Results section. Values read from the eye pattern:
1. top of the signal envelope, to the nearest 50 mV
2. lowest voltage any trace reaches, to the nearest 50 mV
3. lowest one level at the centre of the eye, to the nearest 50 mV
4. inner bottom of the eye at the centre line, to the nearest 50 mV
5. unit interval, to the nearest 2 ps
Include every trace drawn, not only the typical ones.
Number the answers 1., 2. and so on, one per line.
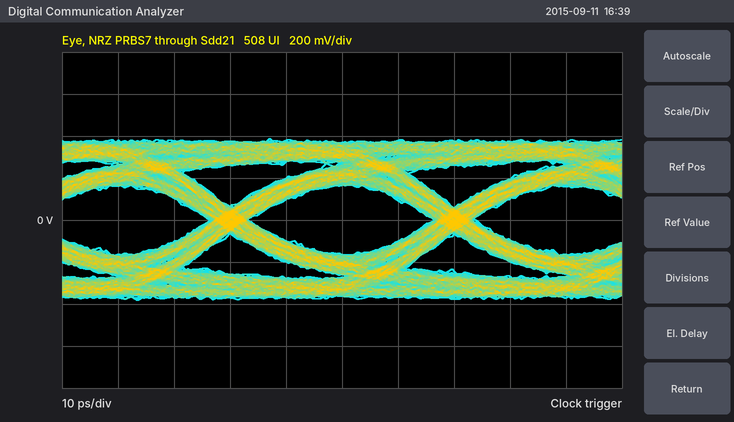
1. 400 mV
2. -400 mV
3. 150 mV
4. -150 mV
5. 40 ps
